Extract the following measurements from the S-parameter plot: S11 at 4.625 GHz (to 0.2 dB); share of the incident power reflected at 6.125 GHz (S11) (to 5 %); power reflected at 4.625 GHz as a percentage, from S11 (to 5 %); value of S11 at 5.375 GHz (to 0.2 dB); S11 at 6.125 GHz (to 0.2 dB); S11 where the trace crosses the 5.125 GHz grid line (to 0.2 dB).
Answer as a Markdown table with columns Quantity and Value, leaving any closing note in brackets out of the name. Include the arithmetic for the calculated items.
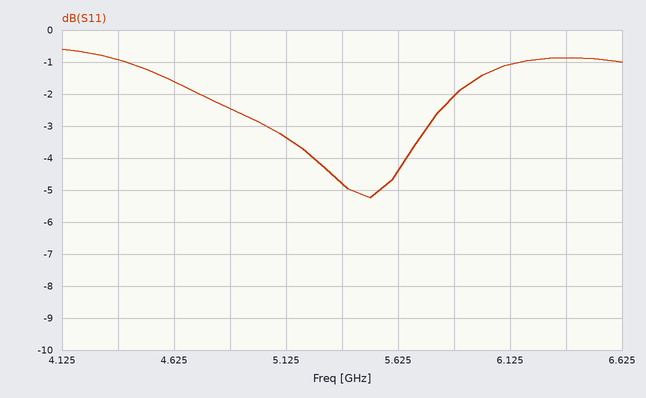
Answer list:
| Quantity | Value |
|---|---|
| S11 at 4.625 GHz | -1.6 dB |
| share of the incident power reflected at 6.125 GHz (S11) | 10^(-1/10) ≈ 79.4 %, so 80 % to the nearest 5 % |
| power reflected at 4.625 GHz as a percentage, from S11 | 10^(-1.6/10) ≈ 69.2 %, so 70 % to the nearest 5 % |
| value of S11 at 5.375 GHz | -4.8 dB |
| S11 at 6.125 GHz | -1.0 dB |
| S11 where the trace crosses the 5.125 GHz grid line | -3.4 dB |
